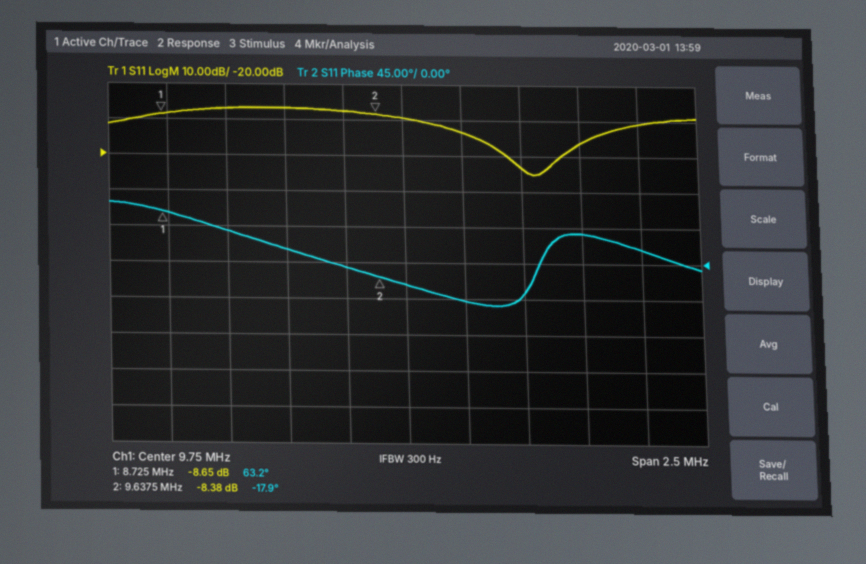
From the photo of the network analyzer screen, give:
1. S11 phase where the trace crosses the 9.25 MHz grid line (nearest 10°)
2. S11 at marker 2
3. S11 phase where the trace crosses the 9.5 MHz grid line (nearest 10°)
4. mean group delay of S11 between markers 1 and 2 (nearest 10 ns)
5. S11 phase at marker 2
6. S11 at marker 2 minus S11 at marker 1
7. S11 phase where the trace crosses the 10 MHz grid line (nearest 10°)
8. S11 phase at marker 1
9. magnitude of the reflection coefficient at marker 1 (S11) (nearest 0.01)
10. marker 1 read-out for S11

20°
-8.38 dB
-10°
250 ns
-17.9°
0.27 dB
-50°
63.2°
0.37
-8.65 dB
